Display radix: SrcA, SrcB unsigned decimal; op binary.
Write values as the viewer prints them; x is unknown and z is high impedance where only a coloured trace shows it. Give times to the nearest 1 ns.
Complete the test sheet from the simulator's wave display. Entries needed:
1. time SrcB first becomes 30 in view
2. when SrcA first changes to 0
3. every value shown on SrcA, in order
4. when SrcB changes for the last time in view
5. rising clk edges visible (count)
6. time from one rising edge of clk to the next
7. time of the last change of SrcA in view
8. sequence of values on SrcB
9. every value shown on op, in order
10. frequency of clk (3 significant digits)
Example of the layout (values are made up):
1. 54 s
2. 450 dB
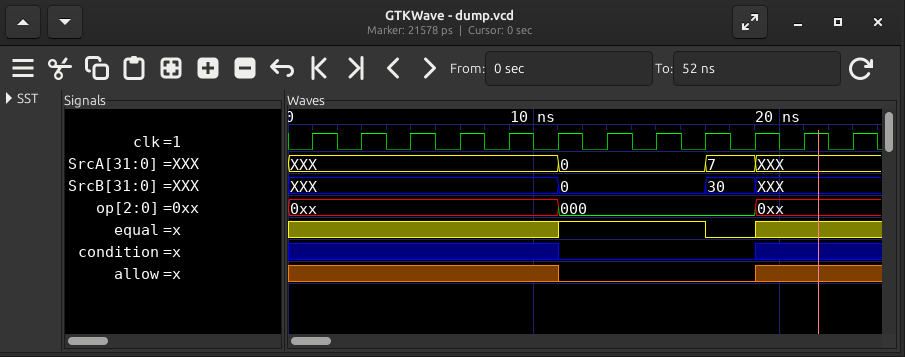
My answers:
1. 17 ns
2. 11 ns
3. XXX, 0, 7, XXX
4. 19 ns
5. 12
6. 2 ns
7. 19 ns
8. XXX, 0, 30, XXX
9. 0xx, 000, 0xx
10. 500 MHz
